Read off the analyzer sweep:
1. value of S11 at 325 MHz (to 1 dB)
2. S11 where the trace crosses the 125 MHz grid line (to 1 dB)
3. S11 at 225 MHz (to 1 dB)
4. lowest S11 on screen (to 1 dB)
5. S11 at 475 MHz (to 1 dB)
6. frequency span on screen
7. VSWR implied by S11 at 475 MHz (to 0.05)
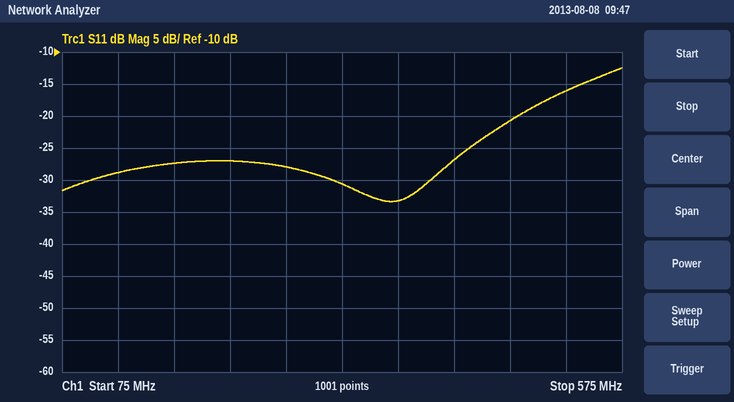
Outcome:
-31 dB
-29 dB
-27 dB
-33 dB
-21 dB
500 MHz
1.20
